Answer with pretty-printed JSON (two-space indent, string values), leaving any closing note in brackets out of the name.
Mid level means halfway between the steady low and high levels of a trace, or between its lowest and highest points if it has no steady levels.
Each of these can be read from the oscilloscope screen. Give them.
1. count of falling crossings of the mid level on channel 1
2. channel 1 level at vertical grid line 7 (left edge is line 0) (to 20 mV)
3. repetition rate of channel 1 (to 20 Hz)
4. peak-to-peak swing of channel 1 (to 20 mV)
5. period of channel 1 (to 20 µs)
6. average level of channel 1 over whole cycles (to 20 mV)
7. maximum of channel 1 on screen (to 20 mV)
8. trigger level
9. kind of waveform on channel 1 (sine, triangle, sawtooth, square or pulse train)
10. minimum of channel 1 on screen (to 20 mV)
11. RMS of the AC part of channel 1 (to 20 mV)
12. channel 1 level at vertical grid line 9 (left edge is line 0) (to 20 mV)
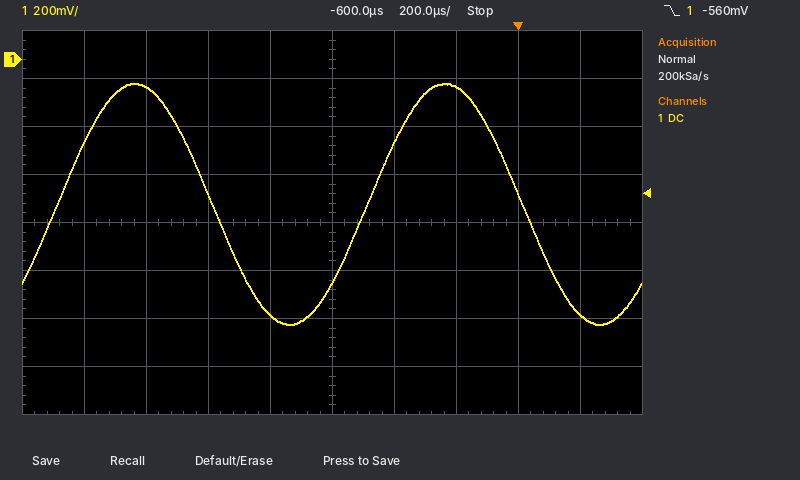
{
  "count of falling crossings of the mid level on channel 1": "2",
  "channel 1 level at vertical grid line 7 (left edge is line 0)": "-120 mV",
  "repetition rate of channel 1": "1.00 kHz",
  "peak-to-peak swing of channel 1": "1.00 V",
  "period of channel 1": "1.00 ms",
  "average level of channel 1 over whole cycles": "-600 mV",
  "maximum of channel 1 on screen": "-100 mV",
  "trigger level": "-560 mV",
  "kind of waveform on channel 1": "sine",
  "minimum of channel 1 on screen": "-1.10 V",
  "RMS of the AC part of channel 1": "360 mV",
  "channel 1 level at vertical grid line 9 (left edge is line 0)": "-1.06 V"
}
